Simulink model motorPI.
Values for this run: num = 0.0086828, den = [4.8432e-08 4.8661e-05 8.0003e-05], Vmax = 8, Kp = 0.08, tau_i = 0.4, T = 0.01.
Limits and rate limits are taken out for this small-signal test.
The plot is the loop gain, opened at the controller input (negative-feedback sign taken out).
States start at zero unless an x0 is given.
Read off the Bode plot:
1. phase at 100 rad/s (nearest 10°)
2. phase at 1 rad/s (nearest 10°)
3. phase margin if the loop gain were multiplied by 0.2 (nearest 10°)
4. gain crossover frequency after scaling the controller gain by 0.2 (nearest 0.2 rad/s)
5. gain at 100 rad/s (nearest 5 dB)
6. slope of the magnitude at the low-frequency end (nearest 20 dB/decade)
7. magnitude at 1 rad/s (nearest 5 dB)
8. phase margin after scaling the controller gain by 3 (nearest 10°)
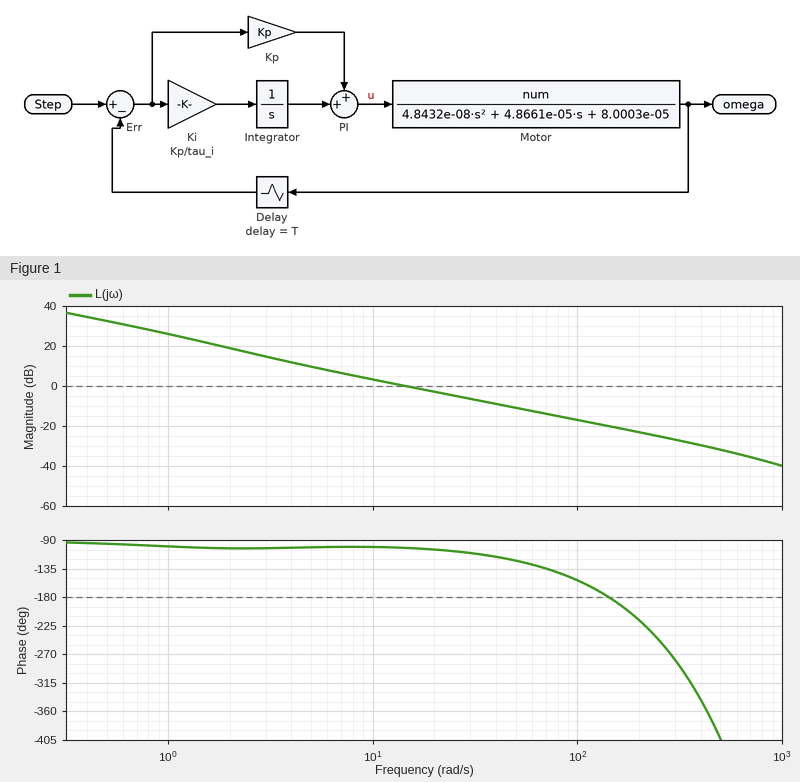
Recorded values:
-150°
-100°
80°
3.2 rad/s
-15 dB
-20 dB/decade
25 dB
60°
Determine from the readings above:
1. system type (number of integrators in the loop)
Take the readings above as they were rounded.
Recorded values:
1
